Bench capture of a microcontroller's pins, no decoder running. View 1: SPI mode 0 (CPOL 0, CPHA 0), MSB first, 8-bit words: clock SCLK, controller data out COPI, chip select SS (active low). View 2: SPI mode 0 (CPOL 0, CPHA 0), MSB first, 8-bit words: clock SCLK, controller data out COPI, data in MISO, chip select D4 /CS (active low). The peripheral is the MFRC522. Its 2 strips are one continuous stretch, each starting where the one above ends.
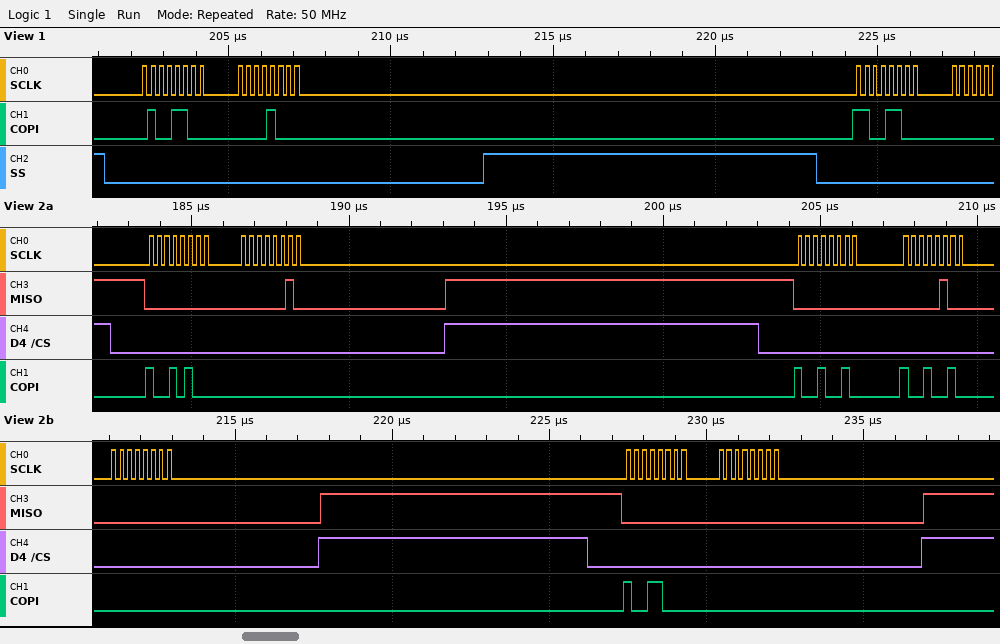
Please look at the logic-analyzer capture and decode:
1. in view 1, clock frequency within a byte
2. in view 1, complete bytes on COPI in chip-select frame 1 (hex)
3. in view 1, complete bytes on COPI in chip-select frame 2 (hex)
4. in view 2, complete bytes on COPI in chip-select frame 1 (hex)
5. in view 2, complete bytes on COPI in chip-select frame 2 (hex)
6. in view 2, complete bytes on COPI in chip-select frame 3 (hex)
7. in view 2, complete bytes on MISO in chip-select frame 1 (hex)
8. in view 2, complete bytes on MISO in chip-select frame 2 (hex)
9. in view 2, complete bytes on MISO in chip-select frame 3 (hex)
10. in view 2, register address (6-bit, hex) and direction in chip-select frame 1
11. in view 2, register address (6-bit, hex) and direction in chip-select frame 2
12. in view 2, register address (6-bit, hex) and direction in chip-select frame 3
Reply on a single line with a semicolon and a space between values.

4 MHz; 0x4C 0x08; 0xCC; 94 00; 92 92 00; 98 00; 00 02; 00 04 00; 00 00; 0x0A read; 0x09 read; 0x0C read
